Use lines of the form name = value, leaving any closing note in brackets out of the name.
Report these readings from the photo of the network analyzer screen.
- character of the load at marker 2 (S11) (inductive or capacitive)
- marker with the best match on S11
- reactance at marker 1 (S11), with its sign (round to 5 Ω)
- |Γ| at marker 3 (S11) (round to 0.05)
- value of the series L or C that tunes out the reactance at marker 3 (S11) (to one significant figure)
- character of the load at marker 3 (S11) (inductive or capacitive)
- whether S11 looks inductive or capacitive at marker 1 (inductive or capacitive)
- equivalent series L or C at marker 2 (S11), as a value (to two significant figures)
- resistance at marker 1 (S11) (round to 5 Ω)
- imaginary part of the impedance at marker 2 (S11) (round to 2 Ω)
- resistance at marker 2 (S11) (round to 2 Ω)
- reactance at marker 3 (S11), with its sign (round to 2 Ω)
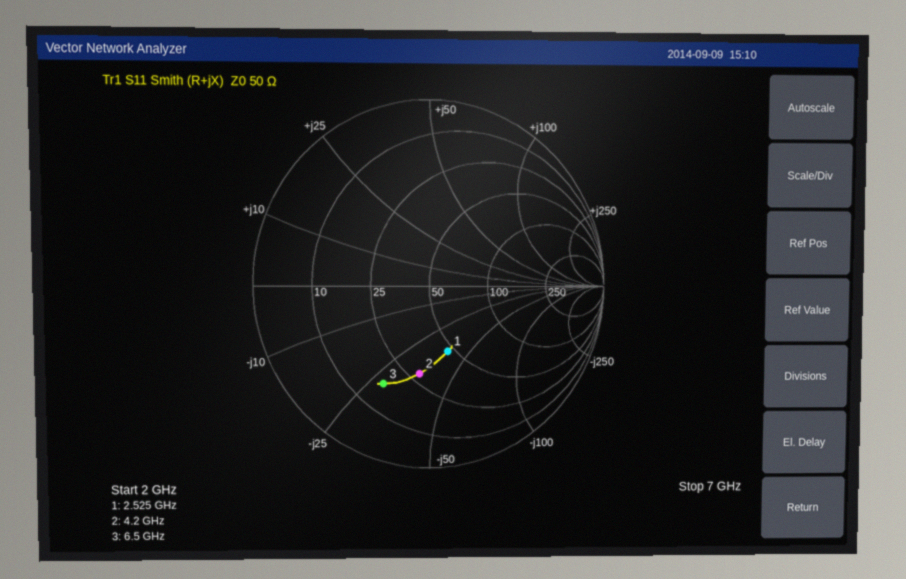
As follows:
character of the load at marker 2 (S11) = capacitive
marker with the best match on S11 = marker 1
reactance at marker 1 (S11), with its sign = -40 Ω
|Γ| at marker 3 (S11) = 0.60
value of the series L or C that tunes out the reactance at marker 3 (S11) = 700 pH
character of the load at marker 3 (S11) = capacitive
whether S11 looks inductive or capacitive at marker 1 = capacitive
equivalent series L or C at marker 2 (S11), as a value = 1.1 pF
resistance at marker 1 (S11) = 45 Ω
imaginary part of the impedance at marker 2 (S11) = -36 Ω
resistance at marker 2 (S11) = 28 Ω
reactance at marker 3 (S11), with its sign = -28 Ω
